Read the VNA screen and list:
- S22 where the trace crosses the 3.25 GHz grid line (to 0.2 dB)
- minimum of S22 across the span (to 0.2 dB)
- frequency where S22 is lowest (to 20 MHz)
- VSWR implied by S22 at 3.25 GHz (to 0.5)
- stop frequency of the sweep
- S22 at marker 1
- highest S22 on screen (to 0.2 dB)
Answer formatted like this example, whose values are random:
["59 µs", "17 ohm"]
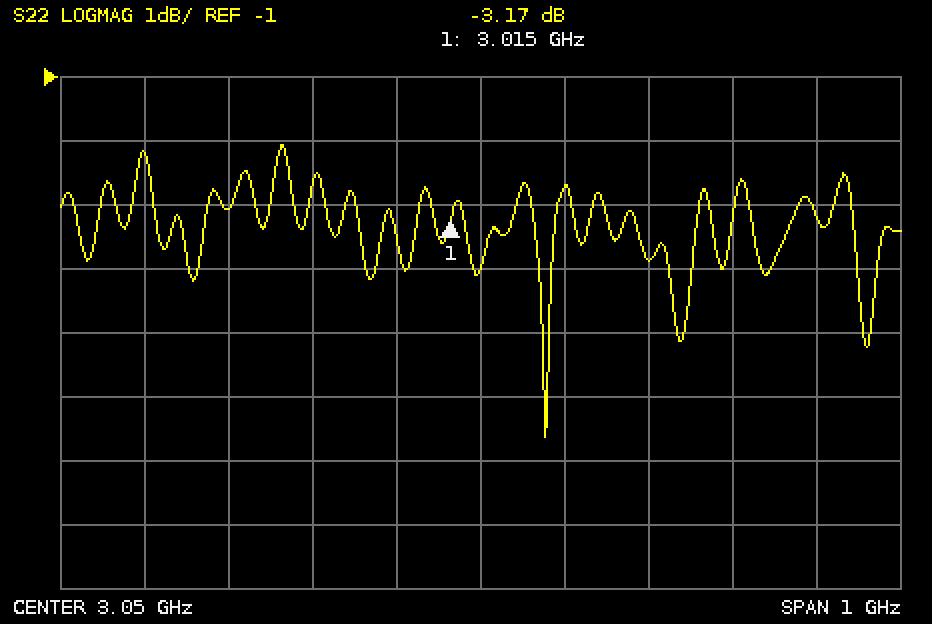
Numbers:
["-3.8 dB", "-6.6 dB", "3.12 GHz", "4.5", "3.55 GHz", "-3.17 dB", "-2.0 dB"]
